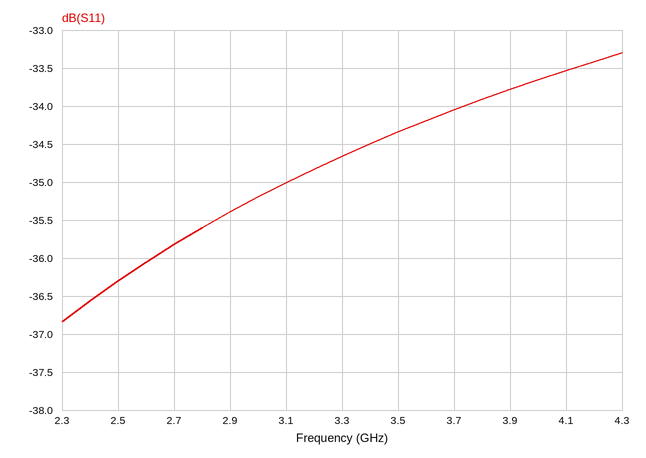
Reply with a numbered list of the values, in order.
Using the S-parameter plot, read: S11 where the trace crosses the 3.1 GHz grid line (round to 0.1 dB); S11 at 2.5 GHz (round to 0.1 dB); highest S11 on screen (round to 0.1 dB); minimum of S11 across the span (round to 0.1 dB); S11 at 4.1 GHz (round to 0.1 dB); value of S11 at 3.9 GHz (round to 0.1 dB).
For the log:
1. -35.0 dB
2. -36.3 dB
3. -33.3 dB
4. -36.8 dB
5. -33.5 dB
6. -33.8 dB
